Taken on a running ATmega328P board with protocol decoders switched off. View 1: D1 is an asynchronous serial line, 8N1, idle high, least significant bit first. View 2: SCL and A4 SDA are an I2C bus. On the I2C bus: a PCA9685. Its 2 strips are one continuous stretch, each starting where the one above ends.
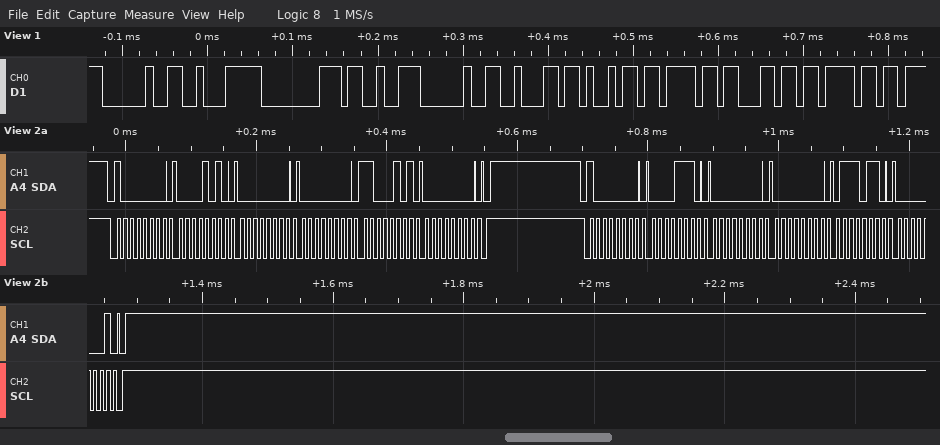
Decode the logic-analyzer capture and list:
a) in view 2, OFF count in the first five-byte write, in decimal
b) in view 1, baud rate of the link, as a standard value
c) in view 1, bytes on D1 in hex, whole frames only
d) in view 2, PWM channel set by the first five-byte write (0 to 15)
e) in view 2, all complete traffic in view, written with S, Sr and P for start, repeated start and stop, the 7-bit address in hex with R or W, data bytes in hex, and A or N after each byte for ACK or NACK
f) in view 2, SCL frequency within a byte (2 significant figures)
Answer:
197
115200 baud
20 E2 80 93 20 62 69 6F 6C 6F
1
S 40W A 0A A 00 A 00 A C5 A 00 A P S 40W A 0E A 00 A 00 A 76 A 01 A P
100 kHz
